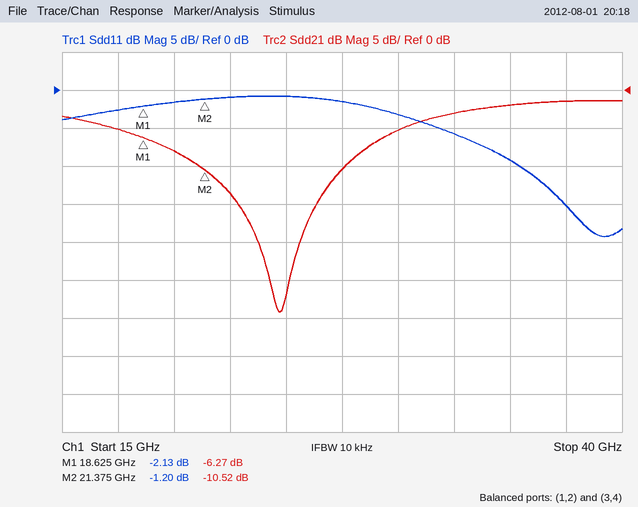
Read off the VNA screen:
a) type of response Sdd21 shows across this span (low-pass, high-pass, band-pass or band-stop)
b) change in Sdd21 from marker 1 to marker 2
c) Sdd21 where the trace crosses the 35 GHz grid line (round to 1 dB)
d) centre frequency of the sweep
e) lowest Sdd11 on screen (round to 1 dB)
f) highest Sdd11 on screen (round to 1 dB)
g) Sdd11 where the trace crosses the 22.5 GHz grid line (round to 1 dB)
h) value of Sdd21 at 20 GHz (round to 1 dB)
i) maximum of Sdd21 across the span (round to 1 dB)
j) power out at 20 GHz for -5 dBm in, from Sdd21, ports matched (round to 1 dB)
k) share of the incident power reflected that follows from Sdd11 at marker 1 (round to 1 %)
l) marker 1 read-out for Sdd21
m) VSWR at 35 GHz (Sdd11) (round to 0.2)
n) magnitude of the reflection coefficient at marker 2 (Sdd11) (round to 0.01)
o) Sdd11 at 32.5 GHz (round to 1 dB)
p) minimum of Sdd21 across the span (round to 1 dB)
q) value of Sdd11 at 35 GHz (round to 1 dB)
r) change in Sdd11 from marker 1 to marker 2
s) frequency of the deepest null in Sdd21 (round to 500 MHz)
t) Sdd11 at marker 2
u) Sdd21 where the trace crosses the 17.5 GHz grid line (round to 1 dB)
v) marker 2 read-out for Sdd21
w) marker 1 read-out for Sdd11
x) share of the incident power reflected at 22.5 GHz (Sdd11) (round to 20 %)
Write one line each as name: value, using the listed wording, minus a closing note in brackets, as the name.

type of response Sdd21 shows across this span: band-stop
change in Sdd21 from marker 1 to marker 2: -4.25 dB
Sdd21 where the trace crosses the 35 GHz grid line: -2 dB
centre frequency of the sweep: 27.5 GHz
lowest Sdd11 on screen: -19 dB
highest Sdd11 on screen: -1 dB
Sdd11 where the trace crosses the 22.5 GHz grid line: -1 dB
value of Sdd21 at 20 GHz: -8 dB
maximum of Sdd21 across the span: -1 dB
power out at 20 GHz for -5 dBm in, from Sdd21, ports matched: -13 dBm
share of the incident power reflected that follows from Sdd11 at marker 1: 61 %
marker 1 read-out for Sdd21: -6.27 dB
VSWR at 35 GHz (Sdd11): 2.0
magnitude of the reflection coefficient at marker 2 (Sdd11): 0.87
Sdd11 at 32.5 GHz: -6 dB
minimum of Sdd21 across the span: -29 dB
value of Sdd11 at 35 GHz: -9 dB
change in Sdd11 from marker 1 to marker 2: 0.93 dB
frequency of the deepest null in Sdd21: 24.5 GHz
Sdd11 at marker 2: -1.20 dB
Sdd21 where the trace crosses the 17.5 GHz grid line: -5 dB
marker 2 read-out for Sdd21: -10.52 dB
marker 1 read-out for Sdd11: -2.13 dB
share of the incident power reflected at 22.5 GHz (Sdd11): 80 %
